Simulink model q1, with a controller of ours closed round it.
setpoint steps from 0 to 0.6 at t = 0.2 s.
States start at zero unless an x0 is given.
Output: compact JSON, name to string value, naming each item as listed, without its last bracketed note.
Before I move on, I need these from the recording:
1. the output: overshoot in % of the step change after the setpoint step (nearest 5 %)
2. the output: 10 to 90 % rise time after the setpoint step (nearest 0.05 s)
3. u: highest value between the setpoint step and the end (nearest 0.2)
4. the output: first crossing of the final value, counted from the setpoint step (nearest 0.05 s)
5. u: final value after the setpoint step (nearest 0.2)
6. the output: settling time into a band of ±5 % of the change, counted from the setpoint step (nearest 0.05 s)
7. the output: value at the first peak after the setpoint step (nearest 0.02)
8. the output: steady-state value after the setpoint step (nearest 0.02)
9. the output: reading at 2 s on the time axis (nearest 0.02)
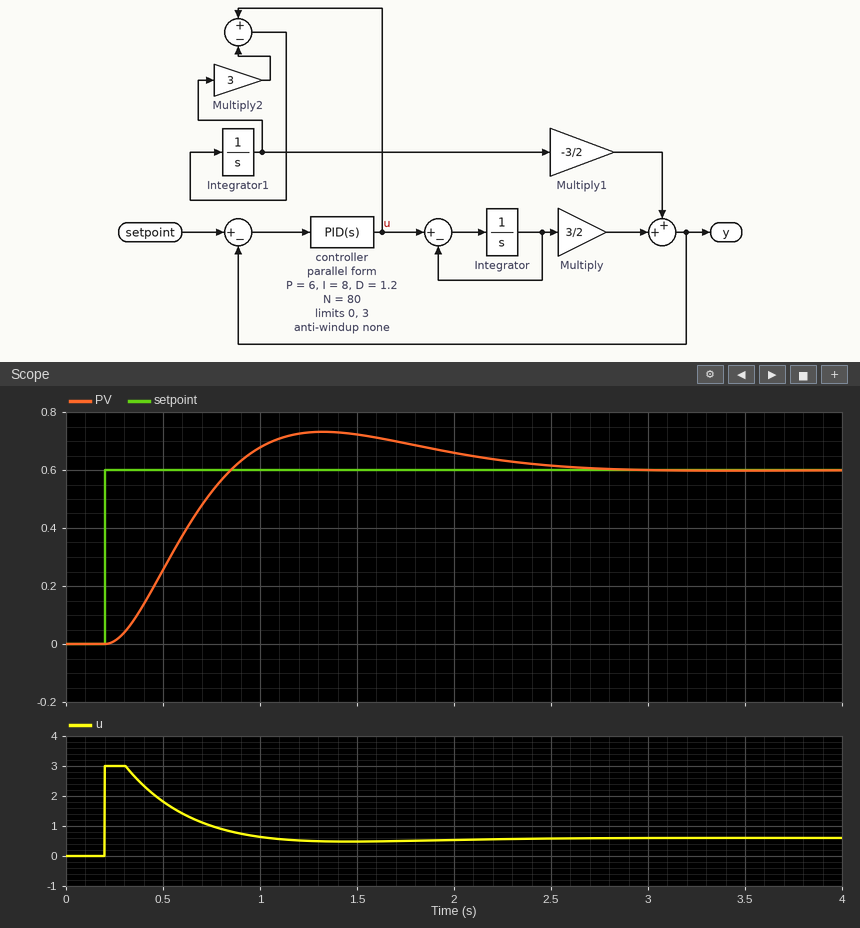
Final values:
{"the output: overshoot in % of the step change after the setpoint step": "20 %", "the output: 10 to 90 % rise time after the setpoint step": "0.45 s", "u: highest value between the setpoint step and the end": "3.0", "the output: first crossing of the final value, counted from the setpoint step": "0.65 s", "u: final value after the setpoint step": "0.6", "the output: settling time into a band of ±5 % of the change, counted from the setpoint step": "2.10 s", "the output: value at the first peak after the setpoint step": "0.74", "the output: steady-state value after the setpoint step": "0.60", "the output: reading at 2 s on the time axis": "0.66"}
